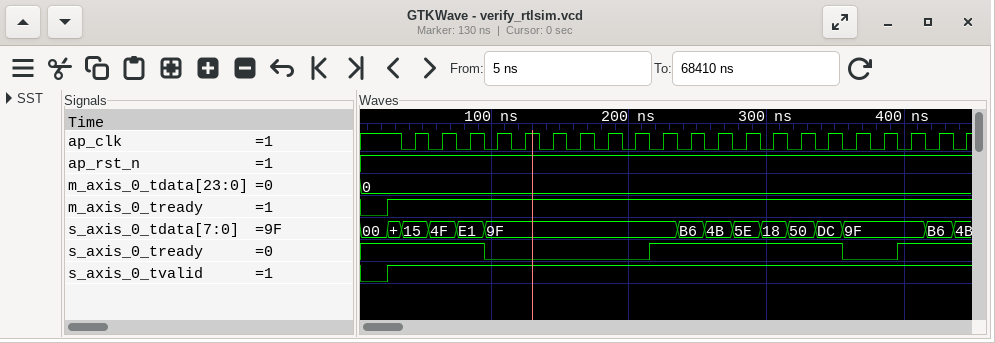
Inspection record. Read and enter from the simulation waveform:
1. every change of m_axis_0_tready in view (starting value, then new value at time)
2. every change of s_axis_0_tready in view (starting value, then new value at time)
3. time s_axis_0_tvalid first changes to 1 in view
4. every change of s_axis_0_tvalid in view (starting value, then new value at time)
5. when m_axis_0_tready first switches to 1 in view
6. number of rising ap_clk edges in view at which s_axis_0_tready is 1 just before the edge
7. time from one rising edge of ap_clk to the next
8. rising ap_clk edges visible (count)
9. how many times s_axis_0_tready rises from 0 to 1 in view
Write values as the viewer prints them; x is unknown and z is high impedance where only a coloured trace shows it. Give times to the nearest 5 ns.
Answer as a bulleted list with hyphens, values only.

- 0, 1 at 25 ns
- 1, 0 at 95 ns, 1 at 215 ns, 0 at 355 ns, 1 at 395 ns
- 25 ns
- 0, 1 at 25 ns
- 25 ns
- 13
- 20 ns
- 21
- 2
